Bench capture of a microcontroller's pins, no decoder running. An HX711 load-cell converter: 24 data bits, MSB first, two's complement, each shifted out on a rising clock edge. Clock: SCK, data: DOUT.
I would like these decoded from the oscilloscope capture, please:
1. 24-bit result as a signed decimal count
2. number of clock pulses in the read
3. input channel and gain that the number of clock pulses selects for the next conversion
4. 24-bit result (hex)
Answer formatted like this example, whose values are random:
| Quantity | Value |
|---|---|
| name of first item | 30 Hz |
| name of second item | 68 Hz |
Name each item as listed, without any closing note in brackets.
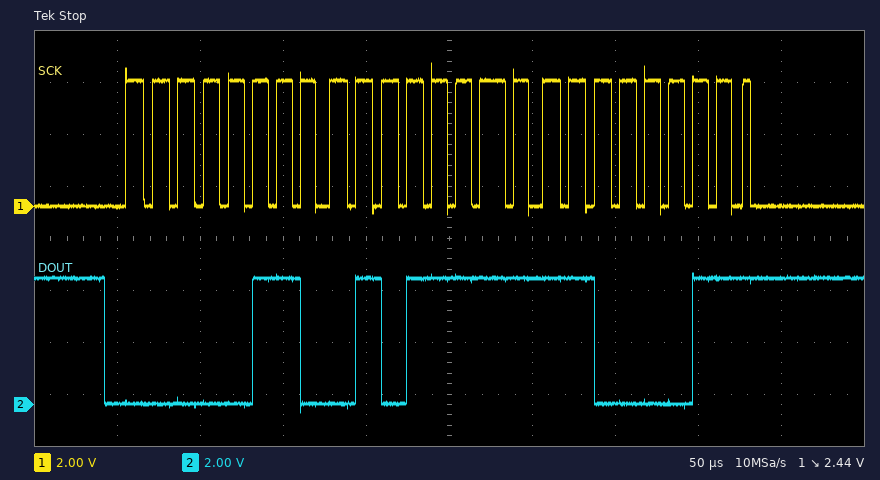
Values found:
| Quantity | Value |
|---|---|
| 24-bit result as a signed decimal count | 417731 |
| number of clock pulses in the read | 25 |
| input channel and gain that the number of clock pulses selects for the next conversion | channel A, gain 128 |
| 24-bit result | 0x065FC3 |
